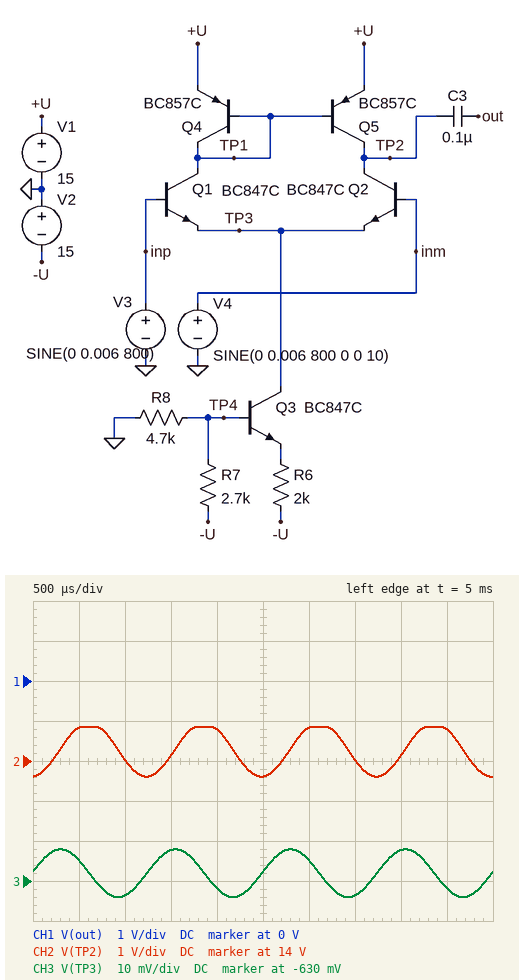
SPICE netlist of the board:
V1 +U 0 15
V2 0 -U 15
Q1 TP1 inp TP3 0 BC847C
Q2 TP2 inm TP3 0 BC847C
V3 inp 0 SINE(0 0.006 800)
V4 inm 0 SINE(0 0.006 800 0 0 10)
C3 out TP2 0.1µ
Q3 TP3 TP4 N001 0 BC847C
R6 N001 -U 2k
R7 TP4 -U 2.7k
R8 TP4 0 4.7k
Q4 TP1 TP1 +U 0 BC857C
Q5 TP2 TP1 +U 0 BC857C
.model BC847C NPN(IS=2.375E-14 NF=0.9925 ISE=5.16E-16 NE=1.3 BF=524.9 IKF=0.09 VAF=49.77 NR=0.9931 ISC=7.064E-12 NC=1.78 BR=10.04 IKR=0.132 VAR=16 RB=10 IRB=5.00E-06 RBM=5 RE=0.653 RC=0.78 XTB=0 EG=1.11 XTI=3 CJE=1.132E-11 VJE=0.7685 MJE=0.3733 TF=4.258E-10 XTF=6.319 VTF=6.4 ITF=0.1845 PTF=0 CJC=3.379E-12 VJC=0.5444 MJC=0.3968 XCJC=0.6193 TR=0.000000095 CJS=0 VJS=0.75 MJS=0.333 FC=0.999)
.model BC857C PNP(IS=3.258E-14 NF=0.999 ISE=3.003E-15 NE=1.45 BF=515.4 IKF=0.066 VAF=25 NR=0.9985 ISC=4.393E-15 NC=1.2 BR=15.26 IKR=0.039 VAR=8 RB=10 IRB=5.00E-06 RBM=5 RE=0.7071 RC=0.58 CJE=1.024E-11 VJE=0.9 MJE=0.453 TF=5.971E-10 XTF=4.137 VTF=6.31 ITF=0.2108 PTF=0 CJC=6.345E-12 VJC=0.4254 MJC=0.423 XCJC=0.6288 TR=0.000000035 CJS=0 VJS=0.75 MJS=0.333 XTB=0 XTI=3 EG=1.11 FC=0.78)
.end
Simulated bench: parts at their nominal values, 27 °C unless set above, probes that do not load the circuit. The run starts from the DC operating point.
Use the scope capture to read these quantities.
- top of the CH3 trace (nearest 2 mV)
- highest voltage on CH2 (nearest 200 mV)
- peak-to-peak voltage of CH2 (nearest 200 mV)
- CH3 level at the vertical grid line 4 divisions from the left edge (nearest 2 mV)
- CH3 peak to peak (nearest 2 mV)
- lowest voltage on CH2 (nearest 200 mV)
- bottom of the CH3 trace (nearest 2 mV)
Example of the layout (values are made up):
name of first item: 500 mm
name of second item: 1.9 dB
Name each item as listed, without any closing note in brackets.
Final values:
top of the CH3 trace: -622 mV
highest voltage on CH2: 14.8 V
peak-to-peak voltage of CH2: 1.2 V
CH3 level at the vertical grid line 4 divisions from the left edge: -632 mV
CH3 peak to peak: 12 mV
lowest voltage on CH2: 13.6 V
bottom of the CH3 trace: -634 mV
